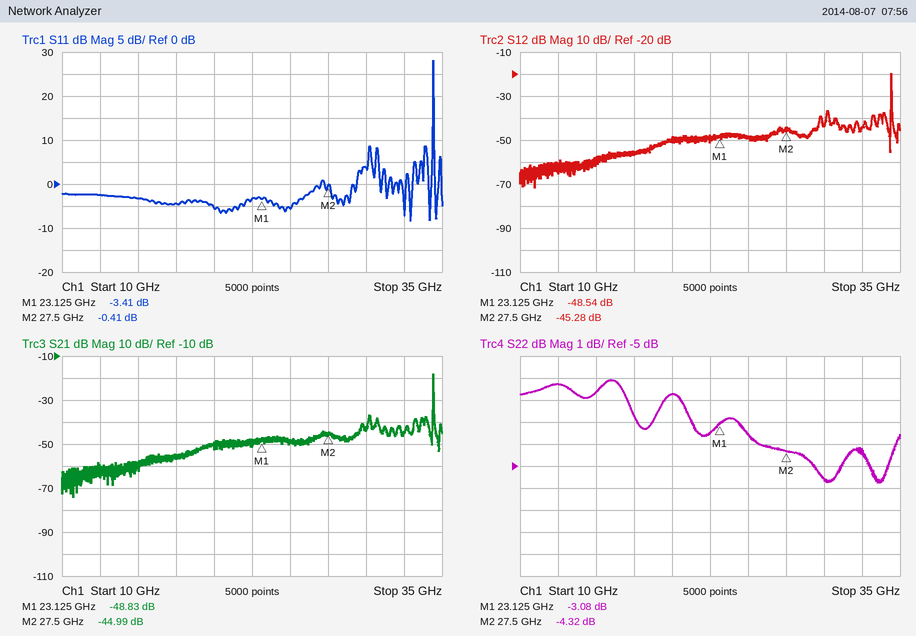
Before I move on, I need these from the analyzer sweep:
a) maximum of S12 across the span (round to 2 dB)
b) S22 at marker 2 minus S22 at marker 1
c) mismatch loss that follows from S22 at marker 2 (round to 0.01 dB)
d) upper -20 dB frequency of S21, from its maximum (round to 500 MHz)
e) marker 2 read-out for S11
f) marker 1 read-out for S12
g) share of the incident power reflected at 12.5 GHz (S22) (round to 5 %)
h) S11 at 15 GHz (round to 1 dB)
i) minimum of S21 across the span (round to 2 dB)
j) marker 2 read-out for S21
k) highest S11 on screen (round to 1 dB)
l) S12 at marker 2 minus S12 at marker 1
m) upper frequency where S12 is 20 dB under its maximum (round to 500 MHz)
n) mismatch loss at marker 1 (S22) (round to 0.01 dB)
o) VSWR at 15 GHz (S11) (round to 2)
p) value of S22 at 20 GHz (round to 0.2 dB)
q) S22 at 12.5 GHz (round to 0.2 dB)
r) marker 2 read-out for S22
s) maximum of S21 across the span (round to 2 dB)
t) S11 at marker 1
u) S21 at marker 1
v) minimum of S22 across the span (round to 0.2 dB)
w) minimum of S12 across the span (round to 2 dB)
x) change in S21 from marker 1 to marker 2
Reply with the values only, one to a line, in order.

-20 dB
-1.24 dB
2.01 dB
34.5 GHz
-0.41 dB
-48.54 dB
75 %
-3 dB
-74 dB
-44.99 dB
28 dB
3.26 dB
34.5 GHz
2.94 dB
6
-1.8 dB
-1.2 dB
-4.32 dB
-18 dB
-3.41 dB
-48.83 dB
-5.8 dB
-72 dB
3.84 dB
